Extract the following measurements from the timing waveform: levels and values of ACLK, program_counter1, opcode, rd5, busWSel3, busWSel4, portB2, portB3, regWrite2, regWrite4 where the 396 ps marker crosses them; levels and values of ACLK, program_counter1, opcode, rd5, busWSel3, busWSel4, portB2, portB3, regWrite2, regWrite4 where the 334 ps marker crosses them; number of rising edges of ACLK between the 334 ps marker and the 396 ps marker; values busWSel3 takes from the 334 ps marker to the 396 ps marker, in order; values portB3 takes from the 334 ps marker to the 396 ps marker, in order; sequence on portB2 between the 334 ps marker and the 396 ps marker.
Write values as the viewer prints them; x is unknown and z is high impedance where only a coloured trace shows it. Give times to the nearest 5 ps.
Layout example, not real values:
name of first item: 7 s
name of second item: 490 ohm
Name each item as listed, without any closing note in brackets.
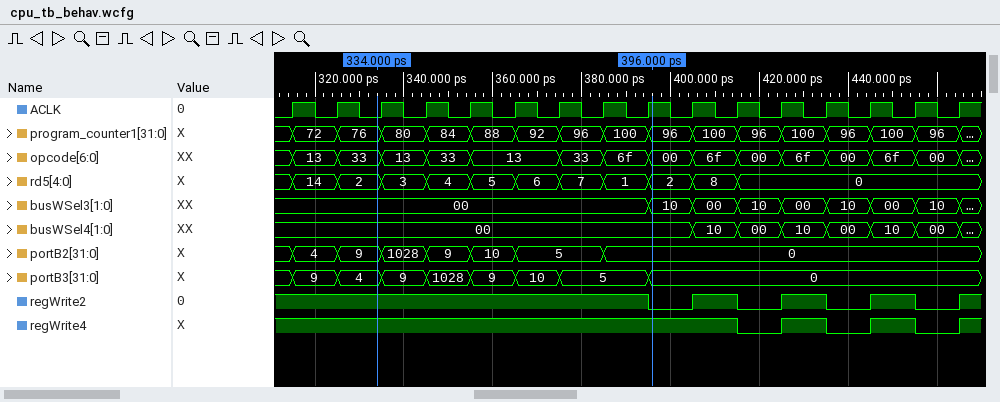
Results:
levels and values of ACLK, program_counter1, opcode, rd5, busWSel3, busWSel4, portB2, portB3, regWrite2, regWrite4 where the 396 ps marker crosses them: ACLK=1, program_counter1=96, opcode=00, rd5=2, busWSel3=10, busWSel4=00, portB2=0, portB3=0, regWrite2=0, regWrite4=1
levels and values of ACLK, program_counter1, opcode, rd5, busWSel3, busWSel4, portB2, portB3, regWrite2, regWrite4 where the 334 ps marker crosses them: ACLK=0, program_counter1=76, opcode=33, rd5=2, busWSel3=00, busWSel4=00, portB2=9, portB3=4, regWrite2=1, regWrite4=1
number of rising edges of ACLK between the 334 ps marker and the 396 ps marker: 7
values busWSel3 takes from the 334 ps marker to the 396 ps marker, in order: 00, 10
values portB3 takes from the 334 ps marker to the 396 ps marker, in order: 4, 9, 1028, 9, 10, 5, 0
sequence on portB2 between the 334 ps marker and the 396 ps marker: 9, 1028, 9, 10, 5, 0
